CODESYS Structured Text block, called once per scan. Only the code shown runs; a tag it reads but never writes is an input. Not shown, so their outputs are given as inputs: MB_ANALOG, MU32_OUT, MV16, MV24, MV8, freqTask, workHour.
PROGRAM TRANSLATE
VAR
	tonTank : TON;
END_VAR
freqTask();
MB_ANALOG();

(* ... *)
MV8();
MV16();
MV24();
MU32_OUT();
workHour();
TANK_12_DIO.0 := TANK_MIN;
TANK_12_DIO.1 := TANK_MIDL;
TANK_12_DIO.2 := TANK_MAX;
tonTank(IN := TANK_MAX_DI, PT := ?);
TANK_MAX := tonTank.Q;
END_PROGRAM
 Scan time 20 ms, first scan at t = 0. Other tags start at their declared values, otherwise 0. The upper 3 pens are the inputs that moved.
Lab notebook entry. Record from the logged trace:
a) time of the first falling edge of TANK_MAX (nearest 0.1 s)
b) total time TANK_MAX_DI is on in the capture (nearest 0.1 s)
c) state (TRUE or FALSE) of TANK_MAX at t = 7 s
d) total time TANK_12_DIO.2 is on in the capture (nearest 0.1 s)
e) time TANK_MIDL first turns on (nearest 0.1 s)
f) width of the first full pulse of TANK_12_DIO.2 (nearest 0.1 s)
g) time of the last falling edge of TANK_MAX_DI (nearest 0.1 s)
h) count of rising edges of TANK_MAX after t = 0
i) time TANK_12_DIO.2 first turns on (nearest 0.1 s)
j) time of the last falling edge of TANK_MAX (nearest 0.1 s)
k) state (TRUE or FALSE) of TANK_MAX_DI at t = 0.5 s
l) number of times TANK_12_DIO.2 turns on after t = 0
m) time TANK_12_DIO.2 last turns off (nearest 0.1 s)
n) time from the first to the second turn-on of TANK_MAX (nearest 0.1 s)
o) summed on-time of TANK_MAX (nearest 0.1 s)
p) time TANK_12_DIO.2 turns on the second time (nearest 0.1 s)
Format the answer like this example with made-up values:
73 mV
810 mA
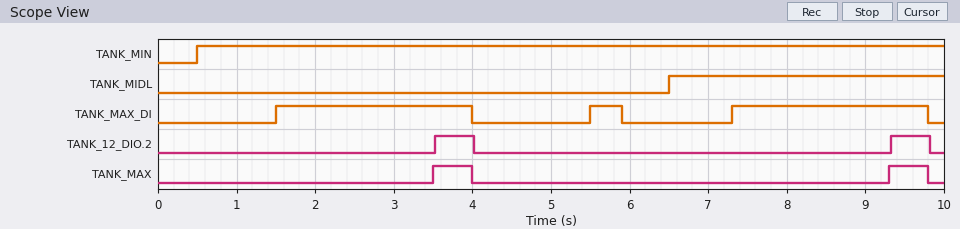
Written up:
4.0 s
5.4 s
FALSE
1.0 s
6.5 s
0.5 s
9.8 s
2
3.5 s
9.8 s
FALSE
2
9.8 s
5.8 s
1.0 s
9.3 s
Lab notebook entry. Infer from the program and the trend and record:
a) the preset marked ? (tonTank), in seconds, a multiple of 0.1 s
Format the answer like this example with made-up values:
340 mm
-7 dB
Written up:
2.0 s
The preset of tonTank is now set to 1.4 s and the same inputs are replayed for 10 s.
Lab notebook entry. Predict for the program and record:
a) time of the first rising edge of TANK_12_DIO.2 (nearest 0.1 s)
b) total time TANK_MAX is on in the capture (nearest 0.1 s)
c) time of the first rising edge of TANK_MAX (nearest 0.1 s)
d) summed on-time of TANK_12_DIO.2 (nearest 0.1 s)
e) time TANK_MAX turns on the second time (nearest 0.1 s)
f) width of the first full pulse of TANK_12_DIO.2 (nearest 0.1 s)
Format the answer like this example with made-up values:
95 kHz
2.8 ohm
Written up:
2.9 s
2.2 s
2.9 s
2.2 s
8.7 s
1.1 s
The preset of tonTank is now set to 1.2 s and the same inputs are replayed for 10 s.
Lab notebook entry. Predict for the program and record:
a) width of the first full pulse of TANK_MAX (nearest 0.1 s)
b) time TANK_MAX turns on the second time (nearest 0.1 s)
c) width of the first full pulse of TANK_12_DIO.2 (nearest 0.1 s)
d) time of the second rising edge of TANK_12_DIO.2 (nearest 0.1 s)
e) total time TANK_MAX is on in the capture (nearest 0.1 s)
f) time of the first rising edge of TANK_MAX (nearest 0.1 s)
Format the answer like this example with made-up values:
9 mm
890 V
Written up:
1.3 s
8.5 s
1.3 s
8.5 s
2.6 s
2.7 s
